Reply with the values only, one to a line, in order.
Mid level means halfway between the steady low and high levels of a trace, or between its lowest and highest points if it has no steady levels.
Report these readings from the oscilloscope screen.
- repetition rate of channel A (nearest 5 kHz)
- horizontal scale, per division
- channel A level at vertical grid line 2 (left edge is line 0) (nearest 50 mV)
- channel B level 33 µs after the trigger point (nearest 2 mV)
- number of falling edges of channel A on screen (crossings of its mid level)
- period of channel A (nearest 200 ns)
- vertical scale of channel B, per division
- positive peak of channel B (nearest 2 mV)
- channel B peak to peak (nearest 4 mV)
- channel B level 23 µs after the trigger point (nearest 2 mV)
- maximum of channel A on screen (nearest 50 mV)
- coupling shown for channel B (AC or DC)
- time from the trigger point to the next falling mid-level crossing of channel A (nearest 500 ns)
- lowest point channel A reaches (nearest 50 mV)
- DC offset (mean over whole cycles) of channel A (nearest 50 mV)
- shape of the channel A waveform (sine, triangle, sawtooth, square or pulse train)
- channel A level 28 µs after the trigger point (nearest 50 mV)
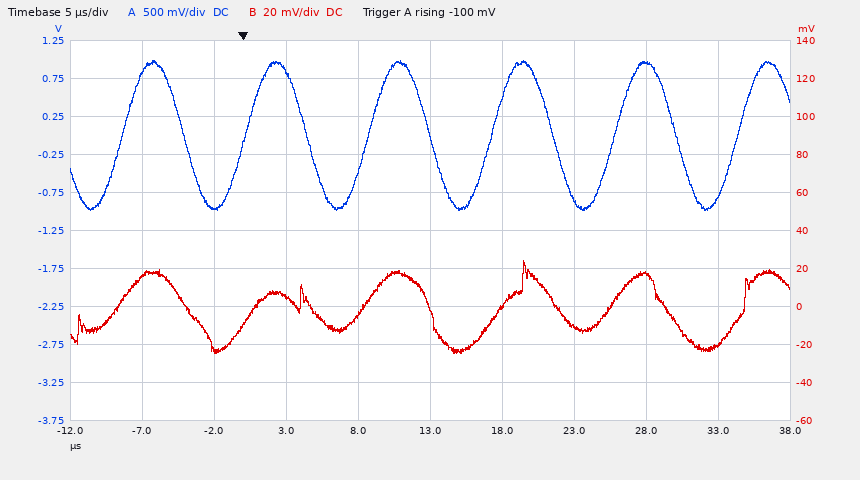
115 kHz
5 µs
-950 mV
-20 mV
5
8.6 µs
20 mV
24 mV
48 mV
-10 mV
1.00 V
DC
4.5 µs
-1.00 V
0 mV
sine
950 mV
